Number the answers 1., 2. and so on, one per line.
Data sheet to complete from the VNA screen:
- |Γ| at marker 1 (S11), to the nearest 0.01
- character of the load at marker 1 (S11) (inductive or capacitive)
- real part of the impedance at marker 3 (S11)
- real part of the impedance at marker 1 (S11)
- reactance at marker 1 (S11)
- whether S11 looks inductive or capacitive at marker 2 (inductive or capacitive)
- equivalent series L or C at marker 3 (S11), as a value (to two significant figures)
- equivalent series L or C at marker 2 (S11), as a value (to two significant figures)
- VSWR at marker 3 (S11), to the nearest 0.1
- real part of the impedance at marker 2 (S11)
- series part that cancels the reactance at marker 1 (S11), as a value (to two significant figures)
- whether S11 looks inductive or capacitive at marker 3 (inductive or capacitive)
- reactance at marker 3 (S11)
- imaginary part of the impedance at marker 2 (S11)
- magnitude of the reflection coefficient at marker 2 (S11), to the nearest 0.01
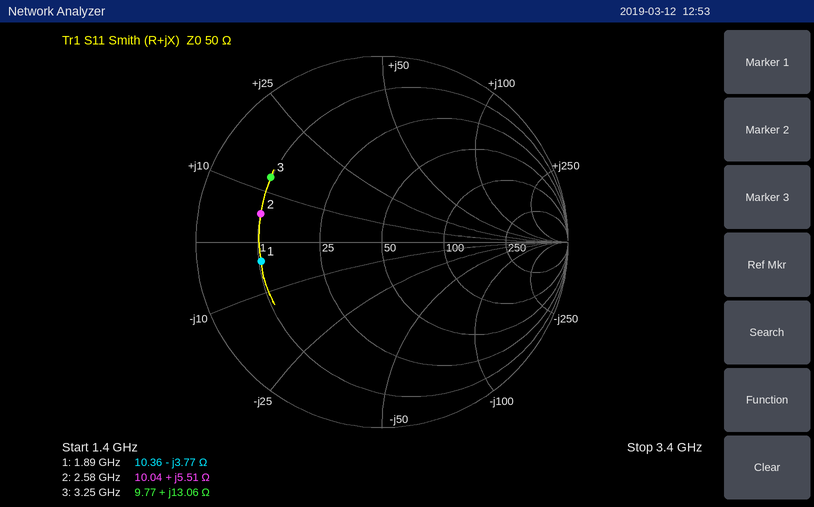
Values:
1. 0.66
2. capacitive
3. 9.77 Ω
4. 10.36 Ω
5. -3.77 Ω
6. inductive
7. 640 pH
8. 340 pH
9. 5.5
10. 10.04 Ω
11. 320 pH
12. inductive
13. +13.06 Ω
14. +5.51 Ω
15. 0.67
